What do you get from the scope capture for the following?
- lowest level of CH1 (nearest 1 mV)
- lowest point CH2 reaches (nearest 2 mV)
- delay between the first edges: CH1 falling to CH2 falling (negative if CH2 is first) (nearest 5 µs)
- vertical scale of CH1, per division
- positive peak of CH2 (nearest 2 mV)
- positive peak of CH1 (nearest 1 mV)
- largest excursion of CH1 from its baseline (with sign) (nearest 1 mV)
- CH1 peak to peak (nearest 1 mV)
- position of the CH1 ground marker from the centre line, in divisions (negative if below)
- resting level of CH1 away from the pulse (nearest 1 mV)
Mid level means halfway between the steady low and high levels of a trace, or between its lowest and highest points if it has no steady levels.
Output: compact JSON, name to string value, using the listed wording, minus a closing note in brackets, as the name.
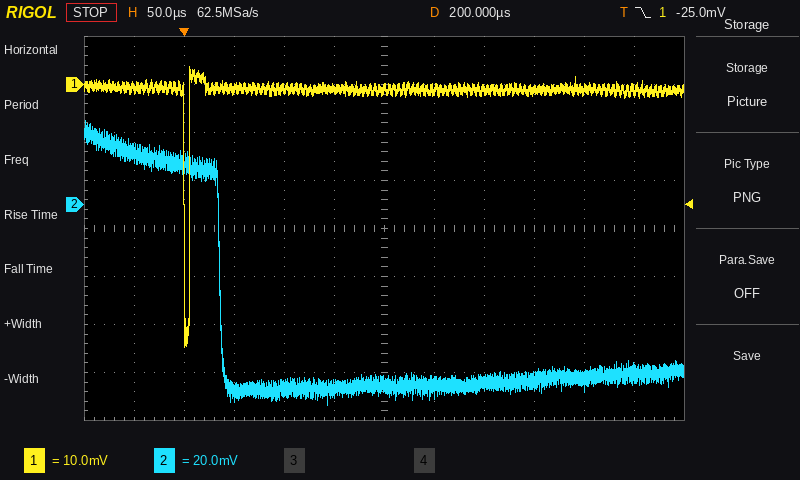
{"lowest level of CH1": "-55 mV", "lowest point CH2 reaches": "-84 mV", "delay between the first edges: CH1 falling to CH2 falling (negative if CH2 is first)": "+35 µs", "vertical scale of CH1, per division": "10 mV", "positive peak of CH2": "36 mV", "positive peak of CH1": "4 mV", "largest excursion of CH1 from its baseline (with sign)": "-54 mV", "CH1 peak to peak": "59 mV", "position of the CH1 ground marker from the centre line, in divisions": "+3.0 div", "resting level of CH1 away from the pulse": "-1 mV"}
